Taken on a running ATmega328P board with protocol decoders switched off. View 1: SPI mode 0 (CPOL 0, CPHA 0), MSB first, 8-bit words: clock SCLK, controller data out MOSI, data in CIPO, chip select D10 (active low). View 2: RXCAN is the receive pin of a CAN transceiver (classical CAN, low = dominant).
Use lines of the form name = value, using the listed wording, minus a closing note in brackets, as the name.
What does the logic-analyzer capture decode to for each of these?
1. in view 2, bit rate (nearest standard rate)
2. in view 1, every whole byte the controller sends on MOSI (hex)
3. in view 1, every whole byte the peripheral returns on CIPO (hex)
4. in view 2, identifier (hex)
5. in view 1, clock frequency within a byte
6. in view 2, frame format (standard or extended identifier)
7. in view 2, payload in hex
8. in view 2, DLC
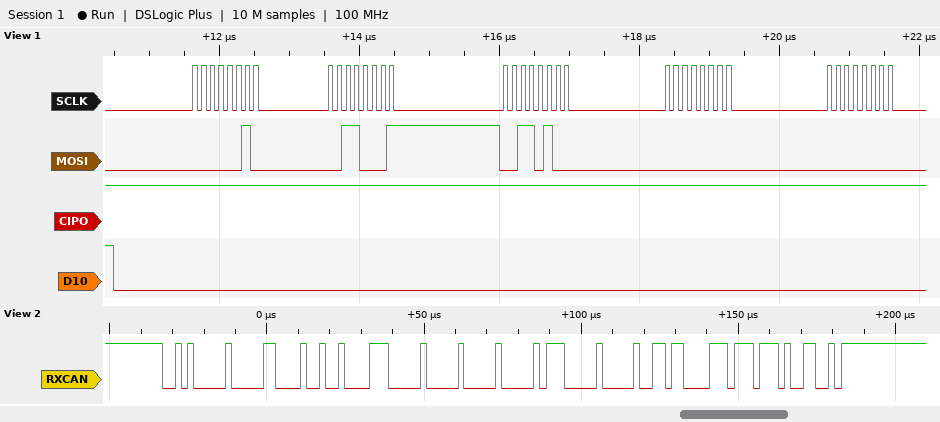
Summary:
in view 2, bit rate = 500 kbit/s
in view 1, every whole byte the controller sends on MOSI = 02 31 34 00 00
in view 1, every whole byte the peripheral returns on CIPO = FF FF FF FF FF
in view 2, identifier = 0x280
in view 1, clock frequency within a byte = 8 MHz
in view 2, frame format = standard
in view 2, payload in hex = 49 0E 00 00 0E 00 1B 0E
in view 2, DLC = 8
